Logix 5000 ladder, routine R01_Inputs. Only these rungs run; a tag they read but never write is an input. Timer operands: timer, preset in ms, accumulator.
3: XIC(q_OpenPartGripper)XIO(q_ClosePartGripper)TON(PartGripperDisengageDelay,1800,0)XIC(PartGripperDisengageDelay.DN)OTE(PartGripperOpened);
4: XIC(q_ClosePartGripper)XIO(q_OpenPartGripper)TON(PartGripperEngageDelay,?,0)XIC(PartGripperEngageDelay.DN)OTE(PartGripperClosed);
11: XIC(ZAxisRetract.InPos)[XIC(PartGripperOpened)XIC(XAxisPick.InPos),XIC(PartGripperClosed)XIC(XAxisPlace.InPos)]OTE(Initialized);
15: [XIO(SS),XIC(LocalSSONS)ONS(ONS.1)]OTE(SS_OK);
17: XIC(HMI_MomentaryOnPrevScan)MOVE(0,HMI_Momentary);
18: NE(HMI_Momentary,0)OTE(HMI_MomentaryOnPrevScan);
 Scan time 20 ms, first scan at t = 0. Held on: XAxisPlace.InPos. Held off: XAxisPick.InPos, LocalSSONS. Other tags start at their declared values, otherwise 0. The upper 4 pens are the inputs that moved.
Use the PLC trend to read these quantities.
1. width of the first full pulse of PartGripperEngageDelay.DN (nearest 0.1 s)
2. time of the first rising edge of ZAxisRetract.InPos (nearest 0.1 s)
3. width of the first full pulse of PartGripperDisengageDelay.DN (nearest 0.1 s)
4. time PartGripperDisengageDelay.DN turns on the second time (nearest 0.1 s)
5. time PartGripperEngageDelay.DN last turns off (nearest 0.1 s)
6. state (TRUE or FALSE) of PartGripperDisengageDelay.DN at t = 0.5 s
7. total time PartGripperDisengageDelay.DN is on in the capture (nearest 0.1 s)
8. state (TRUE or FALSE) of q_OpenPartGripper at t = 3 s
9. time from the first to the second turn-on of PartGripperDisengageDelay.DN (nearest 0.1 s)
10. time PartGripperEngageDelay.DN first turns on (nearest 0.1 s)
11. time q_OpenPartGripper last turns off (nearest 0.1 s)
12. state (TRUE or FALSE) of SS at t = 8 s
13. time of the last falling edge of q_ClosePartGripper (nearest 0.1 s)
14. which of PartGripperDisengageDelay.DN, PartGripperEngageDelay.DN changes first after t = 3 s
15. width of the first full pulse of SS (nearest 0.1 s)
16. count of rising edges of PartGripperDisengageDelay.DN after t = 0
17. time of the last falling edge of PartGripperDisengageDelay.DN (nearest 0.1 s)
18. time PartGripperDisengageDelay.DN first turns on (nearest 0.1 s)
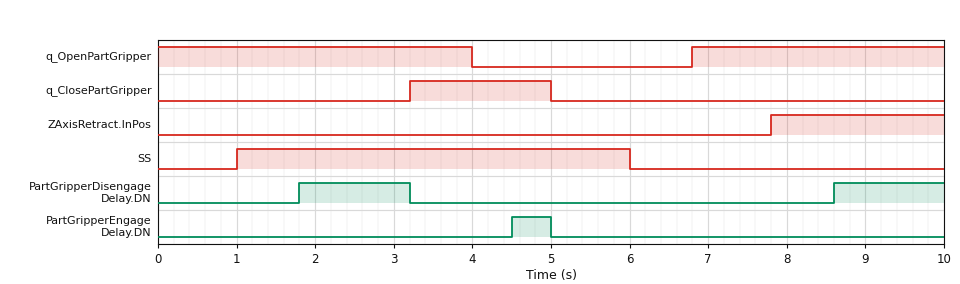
0.5 s
7.8 s
1.4 s
8.6 s
5.0 s
FALSE
2.8 s
TRUE
6.8 s
4.5 s
4.0 s
FALSE
5.0 s
PartGripperDisengageDelay.DN
5.0 s
2
3.2 s
1.8 s
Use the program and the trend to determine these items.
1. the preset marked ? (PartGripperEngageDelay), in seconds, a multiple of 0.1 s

0.5 s
